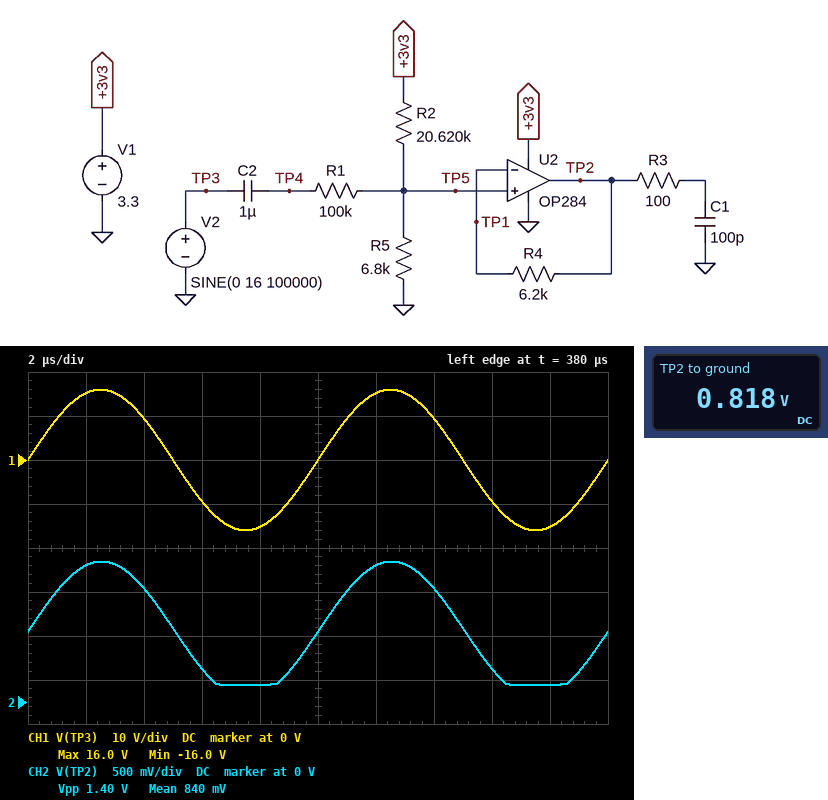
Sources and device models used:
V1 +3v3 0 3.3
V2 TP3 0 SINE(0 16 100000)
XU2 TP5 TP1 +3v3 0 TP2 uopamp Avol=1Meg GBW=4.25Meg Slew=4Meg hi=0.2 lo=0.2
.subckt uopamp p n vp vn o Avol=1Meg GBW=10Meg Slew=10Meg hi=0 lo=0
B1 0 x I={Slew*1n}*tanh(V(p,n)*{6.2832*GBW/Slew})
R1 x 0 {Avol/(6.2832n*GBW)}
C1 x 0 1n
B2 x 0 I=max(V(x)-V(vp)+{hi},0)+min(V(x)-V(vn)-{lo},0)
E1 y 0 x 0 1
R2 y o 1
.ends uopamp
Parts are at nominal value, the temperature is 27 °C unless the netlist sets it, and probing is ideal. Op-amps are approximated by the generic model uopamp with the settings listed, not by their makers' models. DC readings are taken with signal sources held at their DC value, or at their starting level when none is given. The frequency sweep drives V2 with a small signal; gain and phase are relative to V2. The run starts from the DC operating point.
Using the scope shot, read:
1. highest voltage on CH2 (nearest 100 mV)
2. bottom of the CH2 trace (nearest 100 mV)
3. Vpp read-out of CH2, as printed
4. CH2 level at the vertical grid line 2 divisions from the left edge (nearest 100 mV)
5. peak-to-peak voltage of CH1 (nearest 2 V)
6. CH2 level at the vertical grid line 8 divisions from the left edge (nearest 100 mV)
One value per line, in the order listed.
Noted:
1.6 V
200 mV
1.40 V
1.3 V
32 V
400 mV
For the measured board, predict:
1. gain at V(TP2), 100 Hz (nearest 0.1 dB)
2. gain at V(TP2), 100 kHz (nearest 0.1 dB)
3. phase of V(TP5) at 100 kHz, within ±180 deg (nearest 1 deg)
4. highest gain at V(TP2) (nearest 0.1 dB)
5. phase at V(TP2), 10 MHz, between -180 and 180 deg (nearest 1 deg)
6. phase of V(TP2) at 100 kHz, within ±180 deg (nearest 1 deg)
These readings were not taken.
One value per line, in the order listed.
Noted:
-26.3 dB
-26.3 dB
0 deg
-26.3 dB
-67 deg
-1 deg
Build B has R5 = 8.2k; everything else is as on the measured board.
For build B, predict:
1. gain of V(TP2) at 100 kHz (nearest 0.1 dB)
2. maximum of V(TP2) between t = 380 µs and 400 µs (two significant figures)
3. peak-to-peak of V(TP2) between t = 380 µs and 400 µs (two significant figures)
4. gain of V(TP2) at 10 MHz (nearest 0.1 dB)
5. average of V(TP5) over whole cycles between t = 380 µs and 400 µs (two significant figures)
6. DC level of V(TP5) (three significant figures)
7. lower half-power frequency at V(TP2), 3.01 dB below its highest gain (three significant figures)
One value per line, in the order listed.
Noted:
-25.1 dB
1.8 V
1.6 V
-33.3 dB
940 mV
939 mV
1.50 Hz
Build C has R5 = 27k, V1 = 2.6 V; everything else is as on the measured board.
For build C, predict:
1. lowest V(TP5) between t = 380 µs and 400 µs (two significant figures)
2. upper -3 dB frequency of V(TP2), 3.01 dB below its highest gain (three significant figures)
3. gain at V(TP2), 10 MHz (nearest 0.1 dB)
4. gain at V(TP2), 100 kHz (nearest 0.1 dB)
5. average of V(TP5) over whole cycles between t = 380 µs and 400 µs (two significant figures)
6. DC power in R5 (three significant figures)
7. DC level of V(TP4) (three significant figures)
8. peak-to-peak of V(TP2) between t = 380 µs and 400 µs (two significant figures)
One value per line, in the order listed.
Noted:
-200 mV
4.26 MHz
-27.8 dB
-19.6 dB
1.5 V
80.5 µW
1.47 V
2.2 V
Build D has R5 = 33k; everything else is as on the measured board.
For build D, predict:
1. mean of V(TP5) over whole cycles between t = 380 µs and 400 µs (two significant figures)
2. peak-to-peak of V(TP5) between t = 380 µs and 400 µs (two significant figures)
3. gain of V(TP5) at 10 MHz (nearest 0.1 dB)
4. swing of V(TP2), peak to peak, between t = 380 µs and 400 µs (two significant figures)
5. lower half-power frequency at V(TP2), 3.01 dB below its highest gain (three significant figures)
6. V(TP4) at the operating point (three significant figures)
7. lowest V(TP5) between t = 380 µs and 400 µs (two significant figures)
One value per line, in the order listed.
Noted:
2.0 V
3.6 V
-19.0 dB
2.9 V
1.41 Hz
2.03 V
230 mV
